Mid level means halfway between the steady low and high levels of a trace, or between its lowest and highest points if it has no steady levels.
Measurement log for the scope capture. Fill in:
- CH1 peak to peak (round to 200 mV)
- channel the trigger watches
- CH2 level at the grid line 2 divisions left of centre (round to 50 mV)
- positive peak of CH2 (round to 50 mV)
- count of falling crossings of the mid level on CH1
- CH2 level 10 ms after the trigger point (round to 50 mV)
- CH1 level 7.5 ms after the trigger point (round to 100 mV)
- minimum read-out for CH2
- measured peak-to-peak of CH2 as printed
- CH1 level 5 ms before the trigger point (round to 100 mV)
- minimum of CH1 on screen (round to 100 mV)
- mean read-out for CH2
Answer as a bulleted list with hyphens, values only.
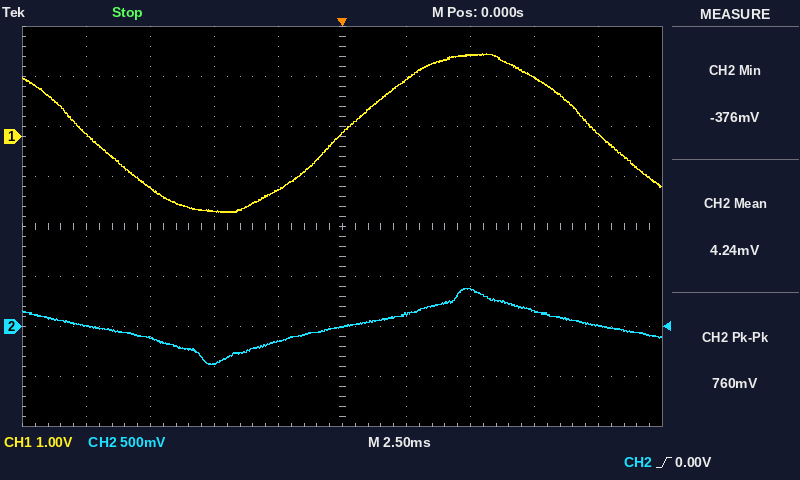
- 3.2 V
- CH2
- -350 mV
- 400 mV
- 2
- 0 mV
- 1.2 V
- -376 mV
- 760 mV
- -1.5 V
- -1.5 V
- 4.24 mV
